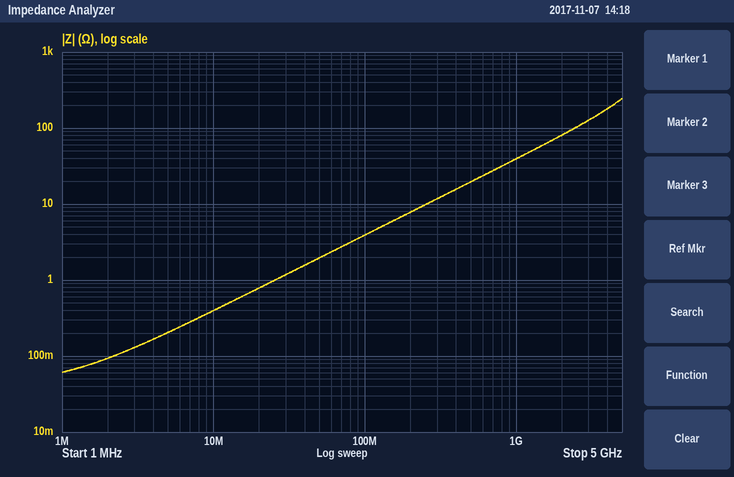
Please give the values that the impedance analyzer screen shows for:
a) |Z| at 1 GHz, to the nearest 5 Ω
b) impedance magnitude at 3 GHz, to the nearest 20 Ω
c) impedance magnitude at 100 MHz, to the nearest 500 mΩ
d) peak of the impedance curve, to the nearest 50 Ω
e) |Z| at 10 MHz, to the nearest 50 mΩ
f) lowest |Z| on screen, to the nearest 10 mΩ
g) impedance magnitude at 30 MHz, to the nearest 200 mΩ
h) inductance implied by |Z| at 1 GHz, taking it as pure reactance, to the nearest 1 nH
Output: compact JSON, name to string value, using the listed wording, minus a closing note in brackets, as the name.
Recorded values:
{"|Z| at 1 GHz, to the nearest 5 Ω": "40 Ω", "impedance magnitude at 3 GHz, to the nearest 20 Ω": "120 Ω", "impedance magnitude at 100 MHz, to the nearest 500 mΩ": "4.0 Ω", "peak of the impedance curve, to the nearest 50 Ω": "250 Ω", "|Z| at 10 MHz, to the nearest 50 mΩ": "400 mΩ", "lowest |Z| on screen, to the nearest 10 mΩ": "60 mΩ", "impedance magnitude at 30 MHz, to the nearest 200 mΩ": "1.2 Ω", "inductance implied by |Z| at 1 GHz, taking it as pure reactance, to the nearest 1 nH": "6 nH"}
